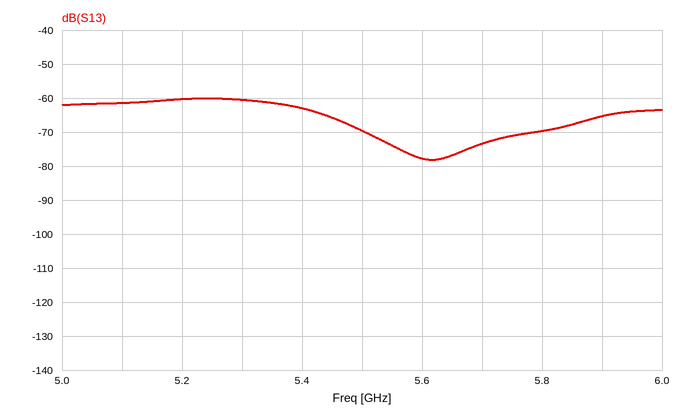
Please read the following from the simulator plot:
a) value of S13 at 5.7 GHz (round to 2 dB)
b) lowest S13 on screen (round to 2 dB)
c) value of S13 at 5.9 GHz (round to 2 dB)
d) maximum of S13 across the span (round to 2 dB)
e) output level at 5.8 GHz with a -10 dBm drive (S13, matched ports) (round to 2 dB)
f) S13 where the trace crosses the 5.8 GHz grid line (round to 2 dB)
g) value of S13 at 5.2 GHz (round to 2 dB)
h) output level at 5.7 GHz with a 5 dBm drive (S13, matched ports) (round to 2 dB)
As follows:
-74 dB
-78 dB
-66 dB
-60 dB
-80 dBm
-70 dB
-60 dB
-68 dBm
